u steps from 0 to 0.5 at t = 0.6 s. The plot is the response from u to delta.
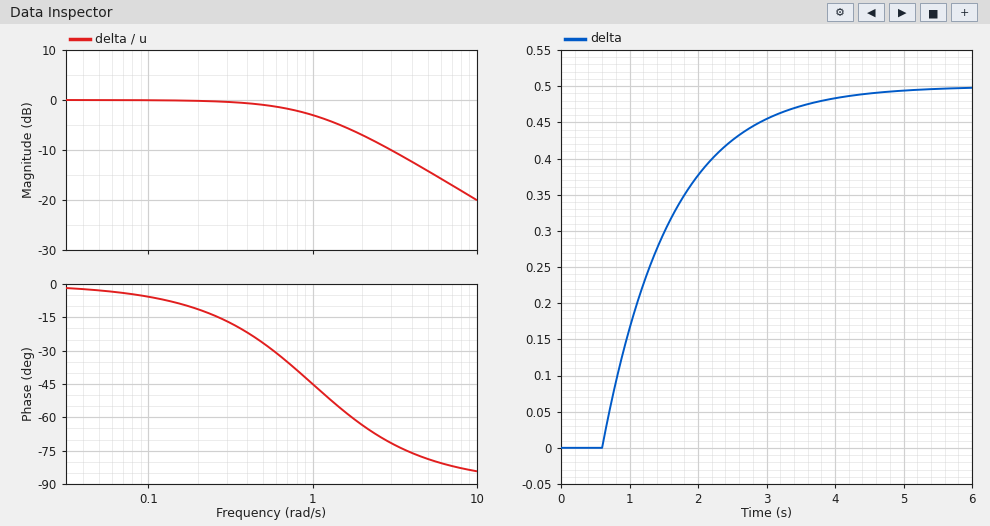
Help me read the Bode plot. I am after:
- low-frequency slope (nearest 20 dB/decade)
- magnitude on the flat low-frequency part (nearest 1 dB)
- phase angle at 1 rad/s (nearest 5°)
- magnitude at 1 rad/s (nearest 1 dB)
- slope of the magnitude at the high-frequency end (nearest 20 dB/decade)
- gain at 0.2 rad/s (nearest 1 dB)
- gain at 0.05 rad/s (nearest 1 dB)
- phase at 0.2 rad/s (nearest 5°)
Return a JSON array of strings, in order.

["0 dB/decade", "0 dB", "-45°", "-3 dB", "-20 dB/decade", "0 dB", "0 dB", "-10°"]
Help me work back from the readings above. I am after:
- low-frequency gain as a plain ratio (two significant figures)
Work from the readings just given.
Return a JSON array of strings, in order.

["1.0"]
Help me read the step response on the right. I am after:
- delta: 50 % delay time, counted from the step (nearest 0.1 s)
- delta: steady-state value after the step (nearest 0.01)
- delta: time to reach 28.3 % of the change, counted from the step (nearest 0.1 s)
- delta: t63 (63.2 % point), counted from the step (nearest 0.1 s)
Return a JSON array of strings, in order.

["0.7 s", "0.50", "0.3 s", "1.0 s"]
